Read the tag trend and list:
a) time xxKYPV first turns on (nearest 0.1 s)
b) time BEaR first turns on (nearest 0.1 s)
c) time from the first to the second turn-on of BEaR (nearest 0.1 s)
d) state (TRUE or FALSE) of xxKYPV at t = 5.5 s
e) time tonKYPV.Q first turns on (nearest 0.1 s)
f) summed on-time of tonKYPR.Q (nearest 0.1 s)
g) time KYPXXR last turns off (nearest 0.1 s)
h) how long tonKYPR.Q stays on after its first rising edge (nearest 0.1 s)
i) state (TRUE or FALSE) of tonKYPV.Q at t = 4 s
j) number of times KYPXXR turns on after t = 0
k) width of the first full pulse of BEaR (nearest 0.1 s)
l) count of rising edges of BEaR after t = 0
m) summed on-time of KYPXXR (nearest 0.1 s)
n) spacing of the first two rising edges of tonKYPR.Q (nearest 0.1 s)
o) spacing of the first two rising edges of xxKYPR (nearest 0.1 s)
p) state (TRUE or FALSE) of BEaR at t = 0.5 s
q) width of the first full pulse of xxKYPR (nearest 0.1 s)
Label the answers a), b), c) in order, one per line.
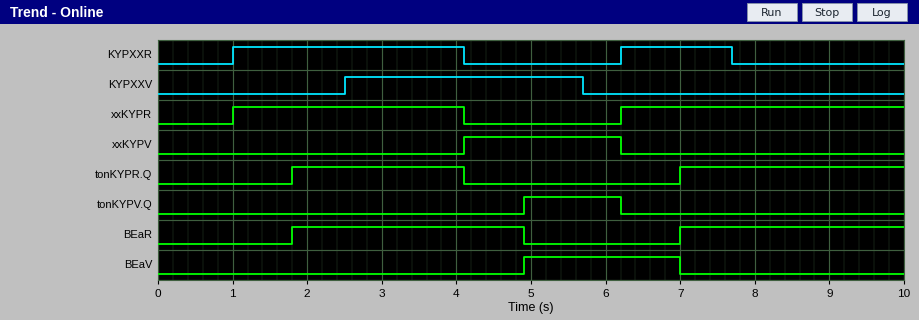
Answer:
a) 4.1 s
b) 1.8 s
c) 5.2 s
d) TRUE
e) 4.9 s
f) 5.3 s
g) 7.7 s
h) 2.3 s
i) FALSE
j) 2
k) 3.1 s
l) 2
m) 4.6 s
n) 5.2 s
o) 5.2 s
p) FALSE
q) 3.1 s
